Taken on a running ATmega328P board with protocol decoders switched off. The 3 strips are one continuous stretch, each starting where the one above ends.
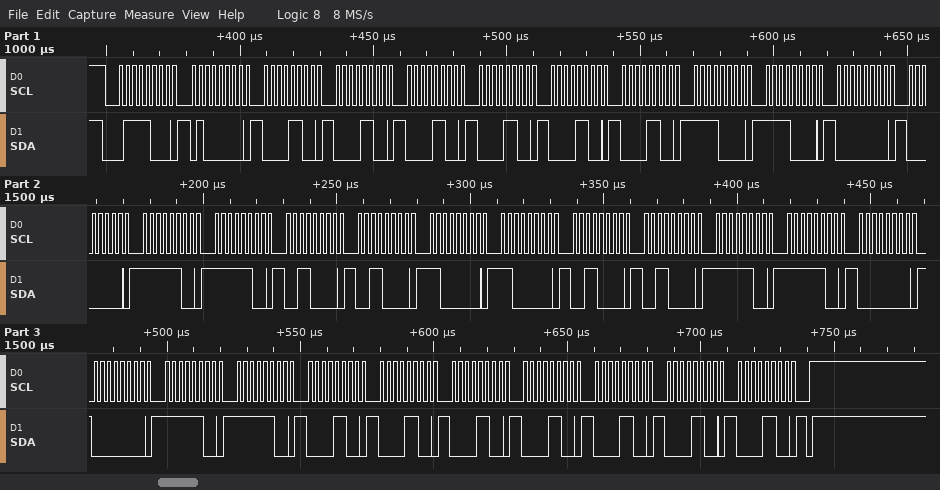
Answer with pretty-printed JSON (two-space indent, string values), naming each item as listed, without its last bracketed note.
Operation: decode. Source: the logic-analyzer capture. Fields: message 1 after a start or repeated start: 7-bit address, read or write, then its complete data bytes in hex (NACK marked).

{
  "message 1 after a start or repeated start: 7-bit address, read or write, then its complete data bytes in hex": "0x3C write: 40 0C 0C 0C 0C 0C 0C F0 F0 00 00 FC FC 30 30 C0 C0 30 30 FC FC 00 00 FC FC 0C 0C 0C 0C 0C 0C 0C"
}
